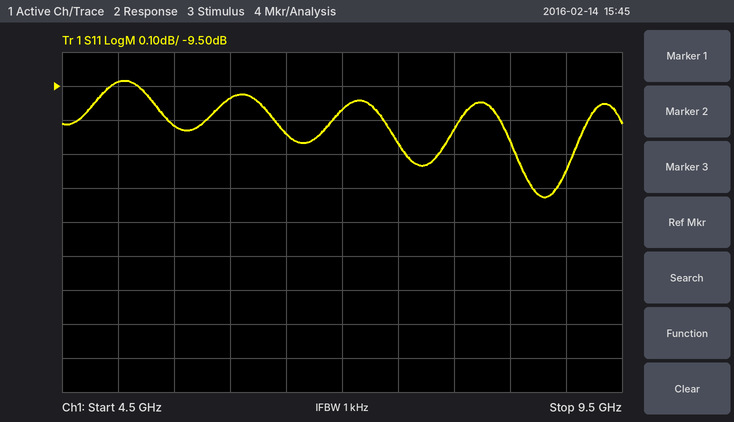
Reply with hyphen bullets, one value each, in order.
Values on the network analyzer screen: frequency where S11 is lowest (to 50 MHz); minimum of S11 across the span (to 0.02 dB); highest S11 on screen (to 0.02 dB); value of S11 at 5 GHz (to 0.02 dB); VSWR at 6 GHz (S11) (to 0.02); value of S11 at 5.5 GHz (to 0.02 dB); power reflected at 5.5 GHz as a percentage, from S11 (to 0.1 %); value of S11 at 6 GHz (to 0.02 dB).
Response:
- 8.80 GHz
- -9.82 dB
- -9.48 dB
- -9.48 dB
- 2.00
- -9.62 dB
- 10.9 %
- -9.54 dB
